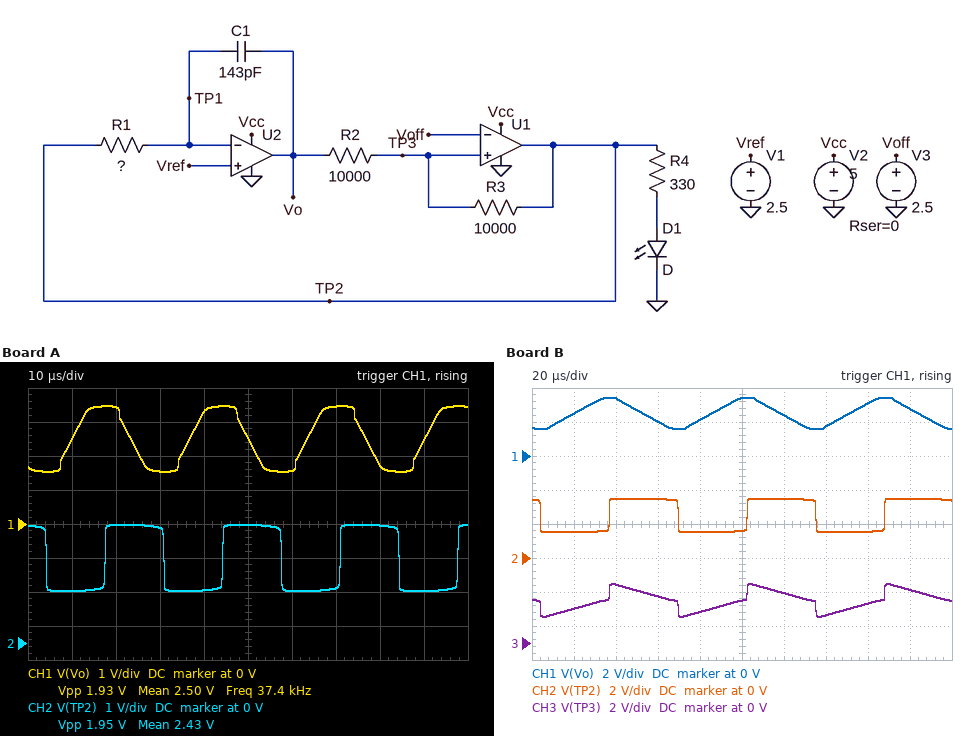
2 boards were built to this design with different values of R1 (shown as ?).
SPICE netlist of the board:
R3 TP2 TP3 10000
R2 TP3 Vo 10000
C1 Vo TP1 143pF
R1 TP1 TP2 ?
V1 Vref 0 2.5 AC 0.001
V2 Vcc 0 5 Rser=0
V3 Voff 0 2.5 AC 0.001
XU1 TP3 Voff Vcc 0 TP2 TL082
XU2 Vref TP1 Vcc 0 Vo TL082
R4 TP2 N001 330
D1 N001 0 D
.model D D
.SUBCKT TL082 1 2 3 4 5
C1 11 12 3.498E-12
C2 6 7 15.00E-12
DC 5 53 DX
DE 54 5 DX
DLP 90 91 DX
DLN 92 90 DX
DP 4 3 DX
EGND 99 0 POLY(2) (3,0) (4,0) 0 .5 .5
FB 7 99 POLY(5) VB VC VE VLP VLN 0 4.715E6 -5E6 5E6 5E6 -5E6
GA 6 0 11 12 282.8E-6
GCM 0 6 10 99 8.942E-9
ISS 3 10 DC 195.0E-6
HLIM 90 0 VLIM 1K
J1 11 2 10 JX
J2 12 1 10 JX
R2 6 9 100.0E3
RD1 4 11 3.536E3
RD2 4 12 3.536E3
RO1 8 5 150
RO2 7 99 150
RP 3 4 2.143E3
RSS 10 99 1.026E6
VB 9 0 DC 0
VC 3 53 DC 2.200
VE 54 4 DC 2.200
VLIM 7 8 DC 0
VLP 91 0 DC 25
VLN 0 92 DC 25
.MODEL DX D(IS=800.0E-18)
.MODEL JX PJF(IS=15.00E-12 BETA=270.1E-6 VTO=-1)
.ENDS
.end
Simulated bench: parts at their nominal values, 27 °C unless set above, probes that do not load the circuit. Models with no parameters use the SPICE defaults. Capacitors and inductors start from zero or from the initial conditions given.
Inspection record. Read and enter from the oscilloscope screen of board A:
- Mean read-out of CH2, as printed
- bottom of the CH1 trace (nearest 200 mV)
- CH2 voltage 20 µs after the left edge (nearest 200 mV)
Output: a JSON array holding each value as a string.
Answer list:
["2.43 V", "1.6 V", "3.4 V"]
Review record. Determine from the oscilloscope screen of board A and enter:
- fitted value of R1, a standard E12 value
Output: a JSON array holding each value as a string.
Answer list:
["27 kΩ"]
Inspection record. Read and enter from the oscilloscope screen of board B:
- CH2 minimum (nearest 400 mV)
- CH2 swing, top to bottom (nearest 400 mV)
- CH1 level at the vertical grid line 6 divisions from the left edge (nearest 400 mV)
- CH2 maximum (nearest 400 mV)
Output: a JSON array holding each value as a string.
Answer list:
["1.6 V", "2.0 V", "2.4 V", "3.6 V"]
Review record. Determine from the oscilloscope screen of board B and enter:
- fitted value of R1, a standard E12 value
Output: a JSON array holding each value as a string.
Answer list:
["100 kΩ"]
